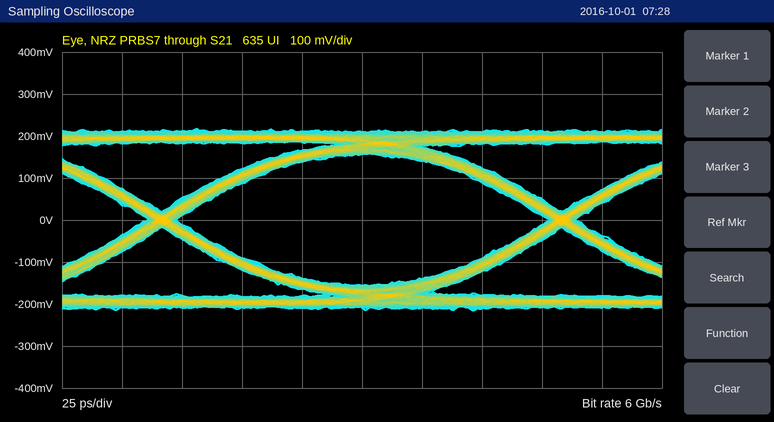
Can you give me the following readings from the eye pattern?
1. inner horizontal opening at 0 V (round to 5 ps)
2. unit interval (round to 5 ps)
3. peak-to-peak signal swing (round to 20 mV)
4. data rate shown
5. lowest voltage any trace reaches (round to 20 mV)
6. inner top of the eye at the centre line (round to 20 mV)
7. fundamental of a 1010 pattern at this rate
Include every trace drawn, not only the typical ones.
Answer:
155 ps
165 ps
440 mV
6 Gb/s
-220 mV
160 mV
3 GHz
